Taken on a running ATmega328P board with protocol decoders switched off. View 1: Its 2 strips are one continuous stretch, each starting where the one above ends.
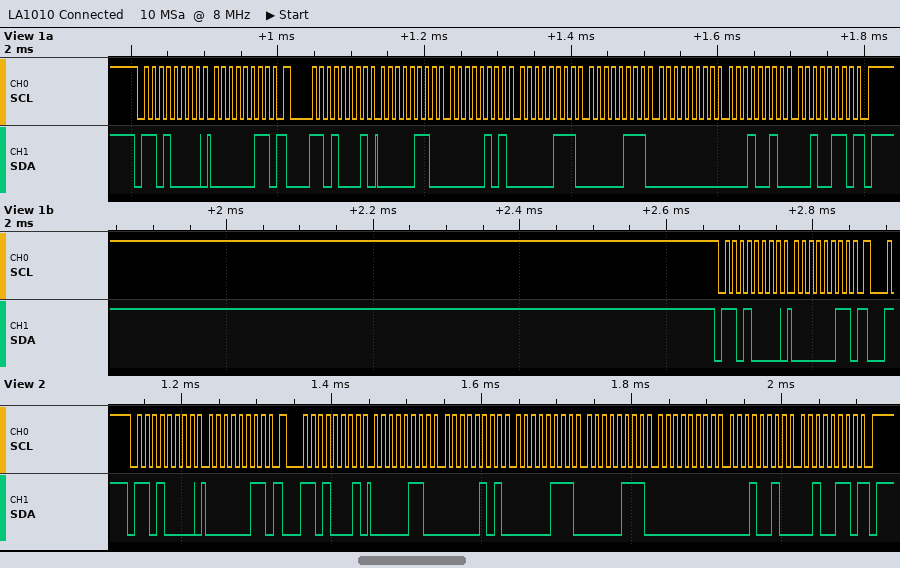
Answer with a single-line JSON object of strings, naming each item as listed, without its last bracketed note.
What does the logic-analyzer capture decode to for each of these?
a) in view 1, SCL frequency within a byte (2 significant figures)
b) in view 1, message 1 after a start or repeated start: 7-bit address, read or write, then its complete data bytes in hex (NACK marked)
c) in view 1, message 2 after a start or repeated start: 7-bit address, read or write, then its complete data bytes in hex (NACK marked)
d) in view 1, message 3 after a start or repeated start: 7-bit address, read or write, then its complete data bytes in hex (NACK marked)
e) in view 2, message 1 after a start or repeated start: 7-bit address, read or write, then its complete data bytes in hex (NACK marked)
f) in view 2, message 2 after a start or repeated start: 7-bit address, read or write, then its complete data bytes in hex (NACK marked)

{"in view 1, SCL frequency within a byte": "100 kHz", "in view 1, message 1 after a start or repeated start: 7-bit address, read or write, then its complete data bytes in hex": "0x68 write: 03", "in view 1, message 2 after a start or repeated start: 7-bit address, read or write, then its complete data bytes in hex": "0x68 read: 06 05 07 07 00 12 26 NACK", "in view 1, message 3 after a start or repeated start: 7-bit address, read or write, then its complete data bytes in hex": "0x68 write: 03", "in view 2, message 1 after a start or repeated start: 7-bit address, read or write, then its complete data bytes in hex": "0x68 write: 03", "in view 2, message 2 after a start or repeated start: 7-bit address, read or write, then its complete data bytes in hex": "0x68 read: 06 05 07 07 00 12 26 NACK"}
